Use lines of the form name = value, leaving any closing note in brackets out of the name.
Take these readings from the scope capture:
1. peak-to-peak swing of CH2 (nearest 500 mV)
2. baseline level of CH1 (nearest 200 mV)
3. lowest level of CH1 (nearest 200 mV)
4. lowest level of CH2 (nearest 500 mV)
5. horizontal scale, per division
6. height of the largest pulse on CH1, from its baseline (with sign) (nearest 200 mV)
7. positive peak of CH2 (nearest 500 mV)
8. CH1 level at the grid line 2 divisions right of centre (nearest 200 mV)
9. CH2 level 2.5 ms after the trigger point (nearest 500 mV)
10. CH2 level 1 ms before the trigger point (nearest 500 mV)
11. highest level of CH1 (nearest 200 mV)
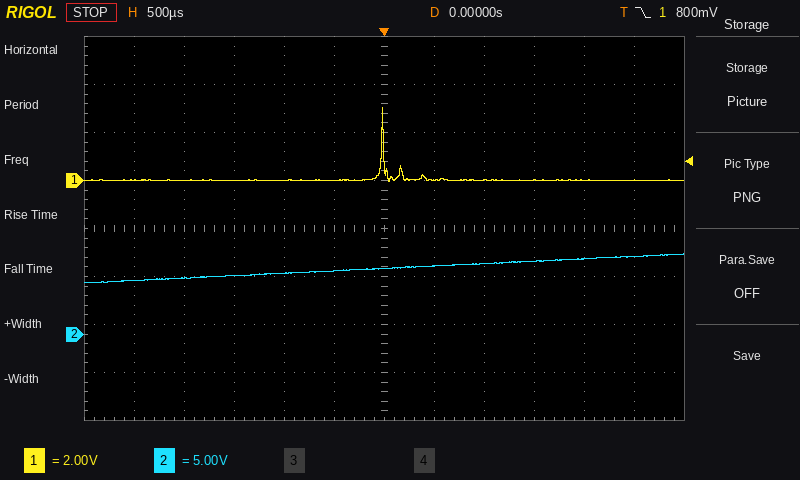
peak-to-peak swing of CH2 = 3.0 V
baseline level of CH1 = 0.0 V
lowest level of CH1 = 0.0 V
lowest level of CH2 = 5.5 V
horizontal scale, per division = 500 µs
height of the largest pulse on CH1, from its baseline (with sign) = +3.0 V
positive peak of CH2 = 8.5 V
CH1 level at the grid line 2 divisions right of centre = 0.0 V
CH2 level 2.5 ms after the trigger point = 8.0 V
CH2 level 1 ms before the trigger point = 6.5 V
highest level of CH1 = 3.0 V
